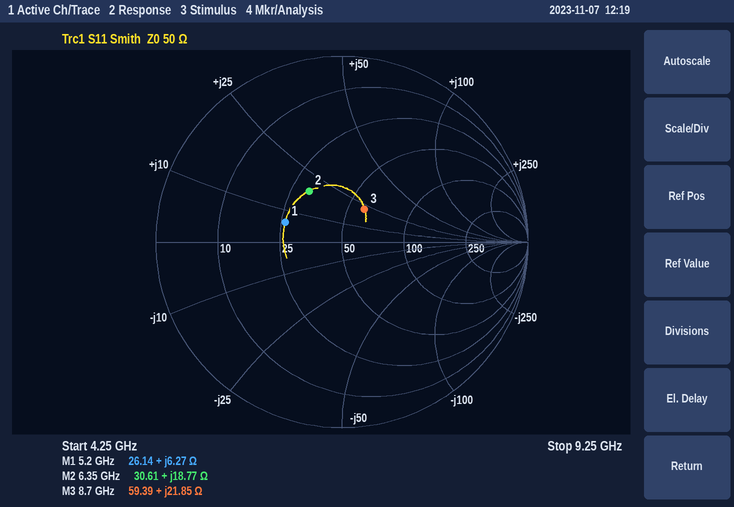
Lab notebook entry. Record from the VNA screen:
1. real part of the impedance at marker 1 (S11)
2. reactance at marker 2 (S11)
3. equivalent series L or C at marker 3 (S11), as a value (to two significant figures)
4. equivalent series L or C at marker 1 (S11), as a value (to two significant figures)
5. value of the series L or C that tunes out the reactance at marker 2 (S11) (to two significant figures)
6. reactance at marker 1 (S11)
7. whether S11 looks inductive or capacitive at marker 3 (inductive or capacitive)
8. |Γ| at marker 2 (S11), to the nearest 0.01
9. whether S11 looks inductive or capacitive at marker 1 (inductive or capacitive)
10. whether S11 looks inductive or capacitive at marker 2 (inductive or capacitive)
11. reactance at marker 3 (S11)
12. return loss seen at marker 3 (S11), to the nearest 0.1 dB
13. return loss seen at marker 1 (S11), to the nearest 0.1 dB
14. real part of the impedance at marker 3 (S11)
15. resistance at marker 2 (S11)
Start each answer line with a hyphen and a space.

- 26.14 Ω
- +18.77 Ω
- 400 pH
- 190 pH
- 1.3 pF
- +6.27 Ω
- inductive
- 0.33
- inductive
- inductive
- +21.85 Ω
- 13.4 dB
- 9.8 dB
- 59.39 Ω
- 30.61 Ω
